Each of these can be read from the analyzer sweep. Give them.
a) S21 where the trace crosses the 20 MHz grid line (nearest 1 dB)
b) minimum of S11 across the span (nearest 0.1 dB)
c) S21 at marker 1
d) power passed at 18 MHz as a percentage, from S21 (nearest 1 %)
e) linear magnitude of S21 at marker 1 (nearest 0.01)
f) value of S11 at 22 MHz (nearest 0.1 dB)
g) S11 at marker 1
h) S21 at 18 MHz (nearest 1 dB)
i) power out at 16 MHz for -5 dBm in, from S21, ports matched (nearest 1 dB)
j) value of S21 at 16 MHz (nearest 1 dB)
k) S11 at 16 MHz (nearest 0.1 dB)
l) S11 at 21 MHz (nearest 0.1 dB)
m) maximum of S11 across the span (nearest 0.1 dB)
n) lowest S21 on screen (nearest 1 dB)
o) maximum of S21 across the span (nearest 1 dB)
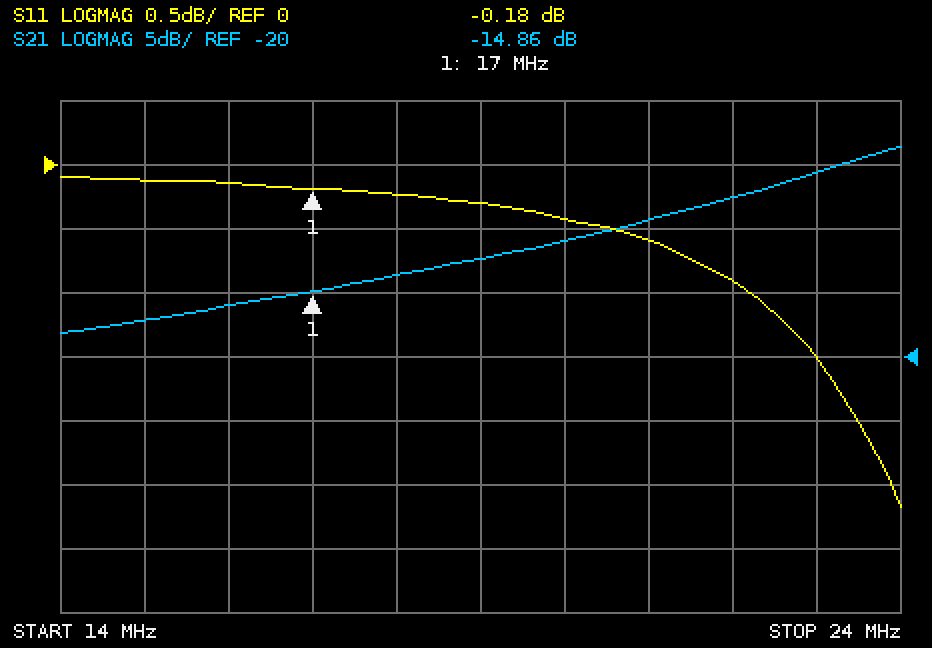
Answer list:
-11 dB
-2.7 dB
-14.86 dB
4 %
0.18
-0.9 dB
-0.18 dB
-14 dB
-21 dBm
-16 dB
-0.1 dB
-0.6 dB
-0.1 dB
-18 dB
-4 dB
